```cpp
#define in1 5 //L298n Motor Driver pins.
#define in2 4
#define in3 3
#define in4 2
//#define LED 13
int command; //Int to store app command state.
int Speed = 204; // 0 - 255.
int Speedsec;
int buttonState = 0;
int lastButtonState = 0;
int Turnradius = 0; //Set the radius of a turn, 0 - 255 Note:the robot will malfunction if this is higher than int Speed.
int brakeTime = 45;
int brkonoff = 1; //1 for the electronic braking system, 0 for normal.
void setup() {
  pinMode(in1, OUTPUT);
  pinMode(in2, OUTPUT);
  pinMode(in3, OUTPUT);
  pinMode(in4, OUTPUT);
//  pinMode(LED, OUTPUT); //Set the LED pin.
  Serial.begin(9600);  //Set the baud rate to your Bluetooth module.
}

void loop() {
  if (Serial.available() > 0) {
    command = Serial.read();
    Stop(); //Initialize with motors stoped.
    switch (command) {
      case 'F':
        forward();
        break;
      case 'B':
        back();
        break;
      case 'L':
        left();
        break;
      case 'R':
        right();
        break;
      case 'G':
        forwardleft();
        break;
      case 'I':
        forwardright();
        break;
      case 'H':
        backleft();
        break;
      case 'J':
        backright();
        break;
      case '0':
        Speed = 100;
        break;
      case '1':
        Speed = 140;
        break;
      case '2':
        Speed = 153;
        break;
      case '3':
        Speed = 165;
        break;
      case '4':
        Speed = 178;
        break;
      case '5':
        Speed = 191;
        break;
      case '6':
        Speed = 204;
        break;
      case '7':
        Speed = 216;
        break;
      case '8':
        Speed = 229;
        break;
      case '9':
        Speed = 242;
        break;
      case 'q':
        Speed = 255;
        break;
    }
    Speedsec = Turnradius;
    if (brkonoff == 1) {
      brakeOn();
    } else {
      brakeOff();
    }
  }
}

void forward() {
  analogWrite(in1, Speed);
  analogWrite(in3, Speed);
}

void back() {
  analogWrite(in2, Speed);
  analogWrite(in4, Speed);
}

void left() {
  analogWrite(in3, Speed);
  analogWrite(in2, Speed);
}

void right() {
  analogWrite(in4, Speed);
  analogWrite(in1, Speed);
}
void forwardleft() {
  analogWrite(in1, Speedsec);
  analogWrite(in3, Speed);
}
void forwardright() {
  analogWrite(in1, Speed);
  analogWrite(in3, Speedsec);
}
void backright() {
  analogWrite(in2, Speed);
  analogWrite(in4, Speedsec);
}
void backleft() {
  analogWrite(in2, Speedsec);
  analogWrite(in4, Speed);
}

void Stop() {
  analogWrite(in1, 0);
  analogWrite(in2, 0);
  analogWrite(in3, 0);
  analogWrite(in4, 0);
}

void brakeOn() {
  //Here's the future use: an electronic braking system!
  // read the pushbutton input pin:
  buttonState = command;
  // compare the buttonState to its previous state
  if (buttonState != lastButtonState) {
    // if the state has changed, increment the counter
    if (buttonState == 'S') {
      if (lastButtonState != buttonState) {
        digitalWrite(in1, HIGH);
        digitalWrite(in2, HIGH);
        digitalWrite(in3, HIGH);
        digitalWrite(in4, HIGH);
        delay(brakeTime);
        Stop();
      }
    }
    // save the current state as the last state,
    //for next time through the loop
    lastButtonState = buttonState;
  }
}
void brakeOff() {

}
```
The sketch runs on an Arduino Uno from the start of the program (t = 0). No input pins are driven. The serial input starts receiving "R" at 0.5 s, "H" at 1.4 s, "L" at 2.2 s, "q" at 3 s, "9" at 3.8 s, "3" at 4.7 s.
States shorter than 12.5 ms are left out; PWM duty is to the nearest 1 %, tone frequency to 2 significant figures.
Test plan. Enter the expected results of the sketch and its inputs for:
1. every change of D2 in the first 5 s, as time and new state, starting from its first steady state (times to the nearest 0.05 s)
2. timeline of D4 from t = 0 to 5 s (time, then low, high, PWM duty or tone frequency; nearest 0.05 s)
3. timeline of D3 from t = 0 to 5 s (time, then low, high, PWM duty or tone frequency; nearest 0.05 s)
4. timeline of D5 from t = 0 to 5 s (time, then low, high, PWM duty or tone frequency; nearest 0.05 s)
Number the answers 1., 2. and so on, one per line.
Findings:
1. 0 s low; 0.5 s high; 2.2 s low
2. 0 s low; 2.2 s high; 3 s low
3. 0 s low; 2.2 s PWM 80 %; 3 s low
4. 0 s low; 0.5 s PWM 80 %; 1.4 s low
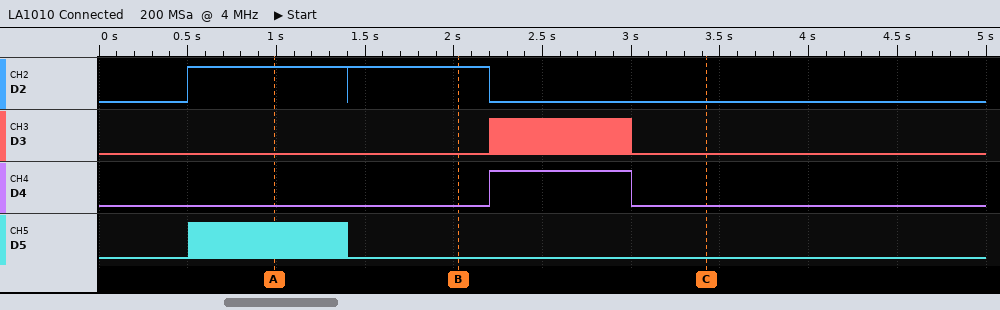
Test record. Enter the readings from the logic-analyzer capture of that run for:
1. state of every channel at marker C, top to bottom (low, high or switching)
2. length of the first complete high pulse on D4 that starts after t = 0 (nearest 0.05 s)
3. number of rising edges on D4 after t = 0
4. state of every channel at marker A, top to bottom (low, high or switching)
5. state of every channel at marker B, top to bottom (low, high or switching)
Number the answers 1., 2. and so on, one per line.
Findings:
1. D2 low, D3 low, D4 low, D5 low
2. 0.80 s
3. 1
4. D2 high, D3 low, D4 low, D5 switching
5. D2 high, D3 low, D4 low, D5 low
